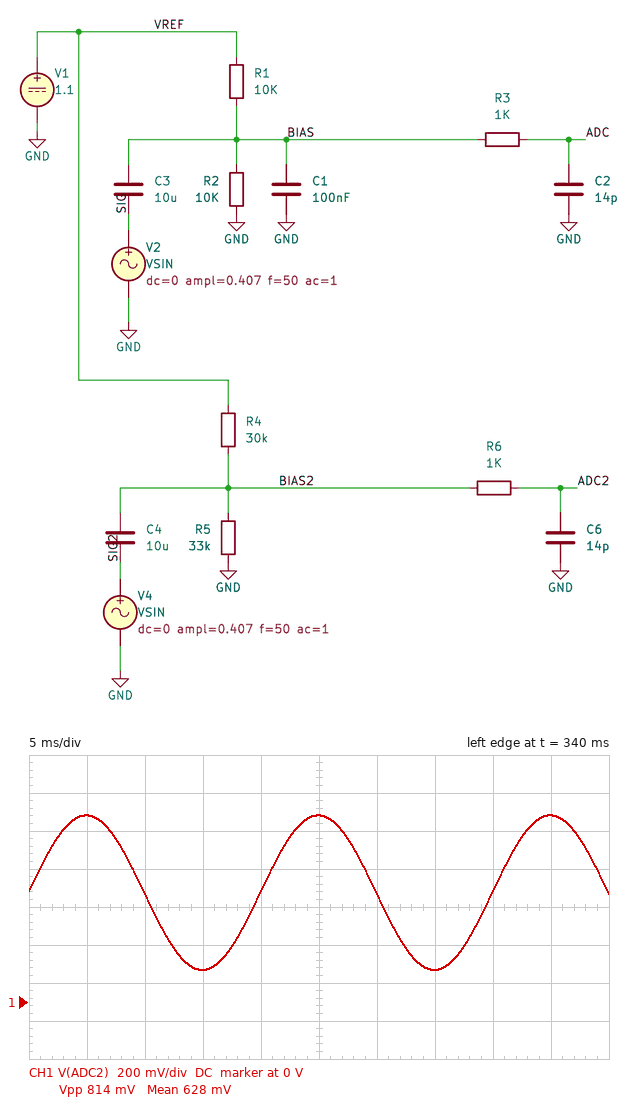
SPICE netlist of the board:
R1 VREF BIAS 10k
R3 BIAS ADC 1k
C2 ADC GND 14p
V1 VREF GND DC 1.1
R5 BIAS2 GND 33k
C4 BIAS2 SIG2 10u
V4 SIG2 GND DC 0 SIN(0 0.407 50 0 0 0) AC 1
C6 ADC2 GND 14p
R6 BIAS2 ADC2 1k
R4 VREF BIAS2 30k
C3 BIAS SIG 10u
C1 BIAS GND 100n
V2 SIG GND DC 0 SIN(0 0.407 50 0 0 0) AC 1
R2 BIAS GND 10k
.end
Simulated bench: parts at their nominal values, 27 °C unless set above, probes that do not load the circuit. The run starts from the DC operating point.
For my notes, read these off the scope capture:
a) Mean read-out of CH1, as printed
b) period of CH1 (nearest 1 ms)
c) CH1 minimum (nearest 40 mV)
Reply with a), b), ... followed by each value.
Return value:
a) 628 mV
b) 20 ms
c) 160 mV
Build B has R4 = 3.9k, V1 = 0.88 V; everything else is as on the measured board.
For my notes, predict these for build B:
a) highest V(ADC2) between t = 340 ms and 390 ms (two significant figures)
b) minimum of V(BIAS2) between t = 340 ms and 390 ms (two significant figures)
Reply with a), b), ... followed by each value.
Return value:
a) 1.2 V
b) 380 mV
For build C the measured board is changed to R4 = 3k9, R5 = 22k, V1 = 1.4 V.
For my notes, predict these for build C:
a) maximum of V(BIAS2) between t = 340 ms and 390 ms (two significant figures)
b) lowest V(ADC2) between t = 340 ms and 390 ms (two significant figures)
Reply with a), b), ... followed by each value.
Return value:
a) 1.6 V
b) 780 mV
